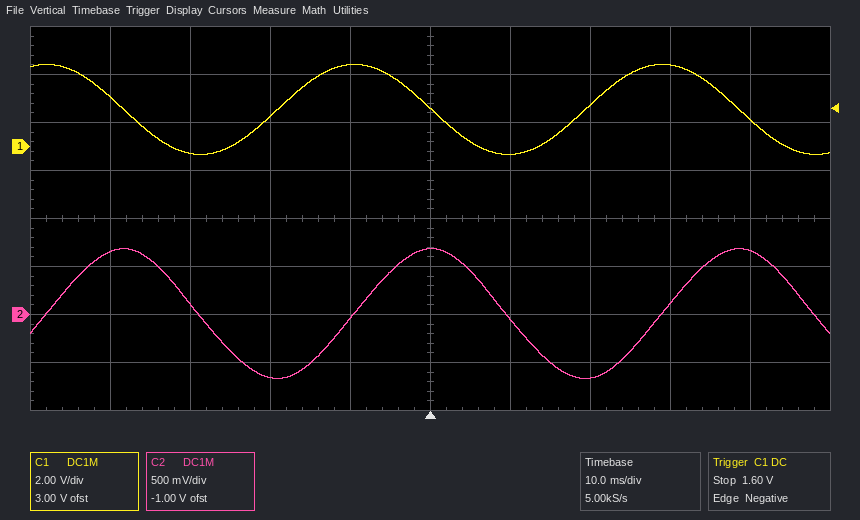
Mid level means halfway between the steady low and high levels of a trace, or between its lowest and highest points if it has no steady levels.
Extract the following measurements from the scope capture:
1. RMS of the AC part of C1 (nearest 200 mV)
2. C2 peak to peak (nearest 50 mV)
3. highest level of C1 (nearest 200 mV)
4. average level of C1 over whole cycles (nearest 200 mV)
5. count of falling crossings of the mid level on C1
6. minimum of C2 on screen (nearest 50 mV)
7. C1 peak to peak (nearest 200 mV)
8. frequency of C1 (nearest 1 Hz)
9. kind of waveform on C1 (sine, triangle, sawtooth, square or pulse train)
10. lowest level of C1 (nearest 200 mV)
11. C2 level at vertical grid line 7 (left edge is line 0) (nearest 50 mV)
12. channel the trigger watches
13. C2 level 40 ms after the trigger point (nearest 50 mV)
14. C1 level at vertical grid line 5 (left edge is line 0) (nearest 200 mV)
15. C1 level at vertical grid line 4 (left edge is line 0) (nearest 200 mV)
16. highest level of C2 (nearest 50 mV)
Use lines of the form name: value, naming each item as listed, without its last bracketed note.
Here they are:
RMS of the AC part of C1: 1.4 V
C2 peak to peak: 1.35 V
highest level of C1: 3.4 V
average level of C1 over whole cycles: 1.6 V
count of falling crossings of the mid level on C1: 3
minimum of C2 on screen: -650 mV
C1 peak to peak: 3.8 V
frequency of C1: 26 Hz
kind of waveform on C1: sine
lowest level of C1: -400 mV
C2 level at vertical grid line 7 (left edge is line 0): -650 mV
channel the trigger watches: C1
C2 level 40 ms after the trigger point: 650 mV
C1 level at vertical grid line 5 (left edge is line 0): 1.6 V
C1 level at vertical grid line 4 (left edge is line 0): 3.4 V
highest level of C2: 700 mV
